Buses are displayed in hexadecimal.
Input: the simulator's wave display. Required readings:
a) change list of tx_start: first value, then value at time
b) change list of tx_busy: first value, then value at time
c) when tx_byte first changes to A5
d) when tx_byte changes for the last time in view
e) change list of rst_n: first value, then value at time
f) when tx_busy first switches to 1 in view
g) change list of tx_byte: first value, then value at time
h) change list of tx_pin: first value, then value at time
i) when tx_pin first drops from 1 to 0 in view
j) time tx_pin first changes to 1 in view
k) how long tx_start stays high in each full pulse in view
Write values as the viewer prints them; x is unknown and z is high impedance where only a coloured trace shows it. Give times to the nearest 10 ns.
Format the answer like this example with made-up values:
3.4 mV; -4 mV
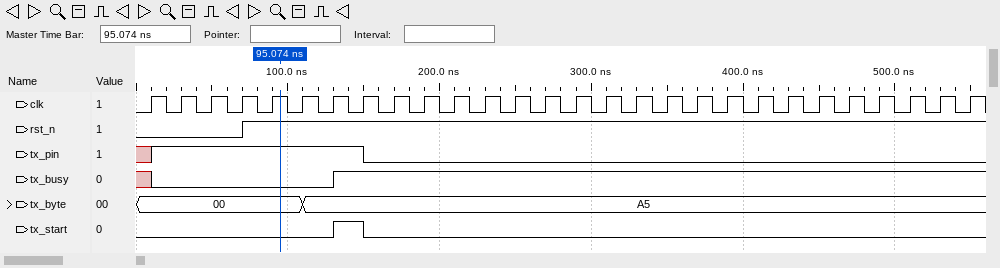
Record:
0, 1 at 130 ns, 0 at 150 ns; x, 0 at 10 ns, 1 at 130 ns; 110 ns; 110 ns; 0, 1 at 70 ns; 130 ns; 00, A5 at 110 ns; x, 1 at 10 ns, 0 at 150 ns; 150 ns; 10 ns; 20 ns
